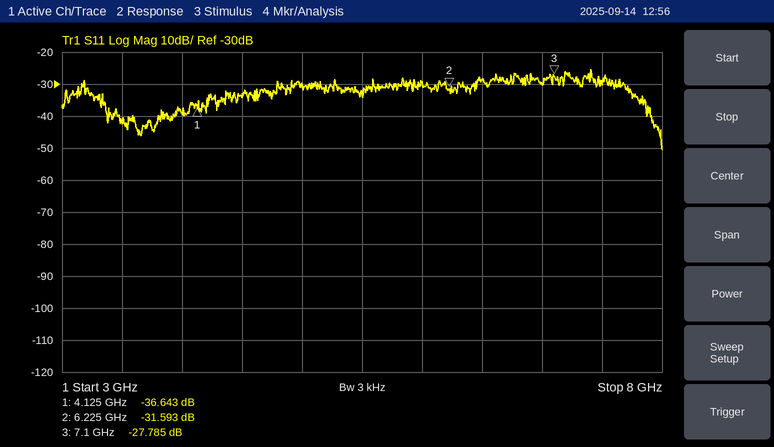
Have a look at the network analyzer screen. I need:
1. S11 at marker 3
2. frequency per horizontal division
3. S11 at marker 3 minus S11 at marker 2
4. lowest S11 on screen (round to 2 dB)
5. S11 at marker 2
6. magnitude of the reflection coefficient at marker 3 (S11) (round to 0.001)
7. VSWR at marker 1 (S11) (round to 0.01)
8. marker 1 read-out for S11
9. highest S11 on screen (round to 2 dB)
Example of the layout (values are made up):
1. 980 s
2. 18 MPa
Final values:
1. -27.785 dB
2. 500 MHz
3. 3.808 dB
4. -50 dB
5. -31.593 dB
6. 0.041
7. 1.03
8. -36.643 dB
9. -26 dB
